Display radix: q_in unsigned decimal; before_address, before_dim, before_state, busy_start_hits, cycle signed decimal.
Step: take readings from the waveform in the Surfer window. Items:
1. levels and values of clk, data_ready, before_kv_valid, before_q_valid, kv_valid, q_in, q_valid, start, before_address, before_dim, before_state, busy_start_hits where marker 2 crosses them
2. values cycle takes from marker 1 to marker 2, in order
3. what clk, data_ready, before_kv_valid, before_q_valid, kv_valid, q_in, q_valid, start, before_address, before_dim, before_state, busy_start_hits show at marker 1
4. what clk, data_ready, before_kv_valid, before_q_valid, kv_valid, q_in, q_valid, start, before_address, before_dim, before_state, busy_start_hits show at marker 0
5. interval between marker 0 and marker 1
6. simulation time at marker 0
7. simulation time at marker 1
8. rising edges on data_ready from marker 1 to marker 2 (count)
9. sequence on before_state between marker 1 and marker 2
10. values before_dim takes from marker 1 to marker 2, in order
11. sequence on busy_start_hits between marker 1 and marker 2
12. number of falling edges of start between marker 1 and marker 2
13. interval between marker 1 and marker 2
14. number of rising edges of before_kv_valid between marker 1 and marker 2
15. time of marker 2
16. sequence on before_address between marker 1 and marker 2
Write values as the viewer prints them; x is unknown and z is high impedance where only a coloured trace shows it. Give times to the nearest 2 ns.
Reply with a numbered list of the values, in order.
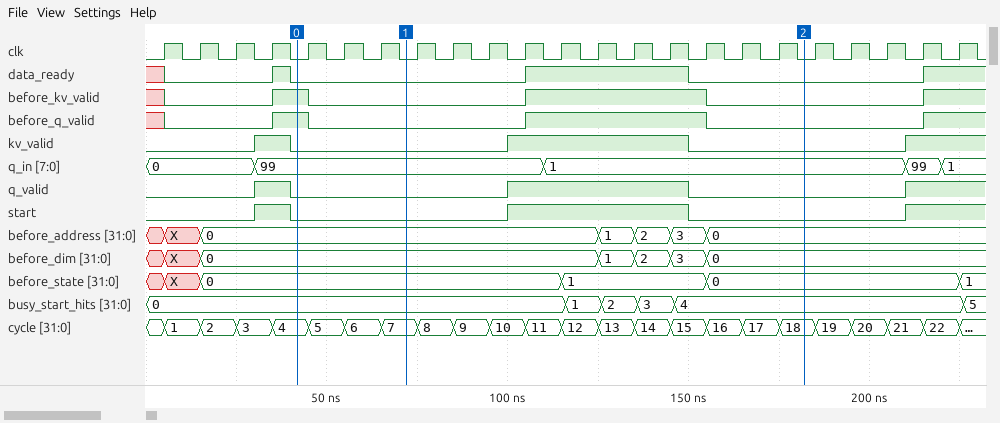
1. clk=0, data_ready=0, before_kv_valid=0, before_q_valid=0, kv_valid=0, q_in=1, q_valid=0, start=0, before_address=0, before_dim=0, before_state=0, busy_start_hits=4
2. 7, 8, 9, 10, 11, 12, 13, 14, 15, 16, 17, 18
3. clk=0, data_ready=0, before_kv_valid=0, before_q_valid=0, kv_valid=0, q_in=99, q_valid=0, start=0, before_address=0, before_dim=0, before_state=0, busy_start_hits=0
4. clk=0, data_ready=0, before_kv_valid=1, before_q_valid=1, kv_valid=0, q_in=99, q_valid=0, start=0, before_address=0, before_dim=0, before_state=0, busy_start_hits=0
5. 30 ns
6. 42 ns
7. 72 ns
8. 1
9. 0, 1, 0
10. 0, 1, 2, 3, 0
11. 0, 1, 2, 3, 4
12. 1
13. 110 ns
14. 1
15. 182 ns
16. 0, 1, 2, 3, 0
